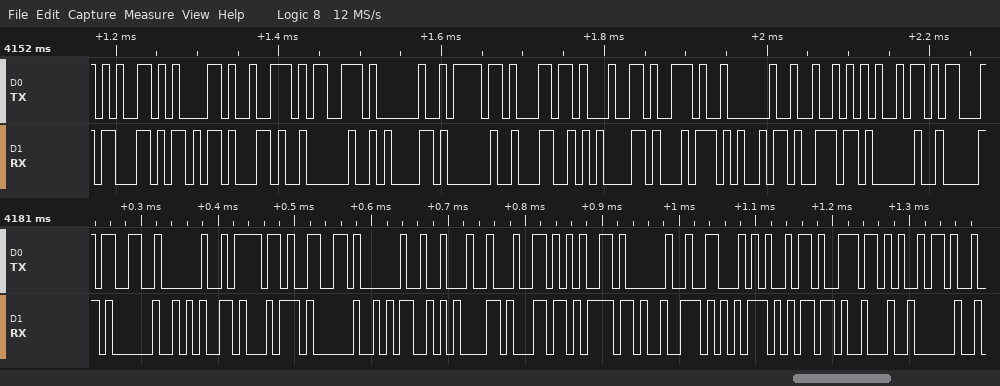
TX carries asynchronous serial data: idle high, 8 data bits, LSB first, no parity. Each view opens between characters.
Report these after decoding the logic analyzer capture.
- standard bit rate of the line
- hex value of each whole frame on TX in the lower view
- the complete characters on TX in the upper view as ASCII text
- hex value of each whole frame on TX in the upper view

115200 baud
33, 20, 6F, 66, 20, 22, 64, 65, 20, 46, 69, 6E, 69
"ears old. Ri"
65, 61, 72, 73, 20, 6F, 6C, 64, 2E, 20, 52, 69
